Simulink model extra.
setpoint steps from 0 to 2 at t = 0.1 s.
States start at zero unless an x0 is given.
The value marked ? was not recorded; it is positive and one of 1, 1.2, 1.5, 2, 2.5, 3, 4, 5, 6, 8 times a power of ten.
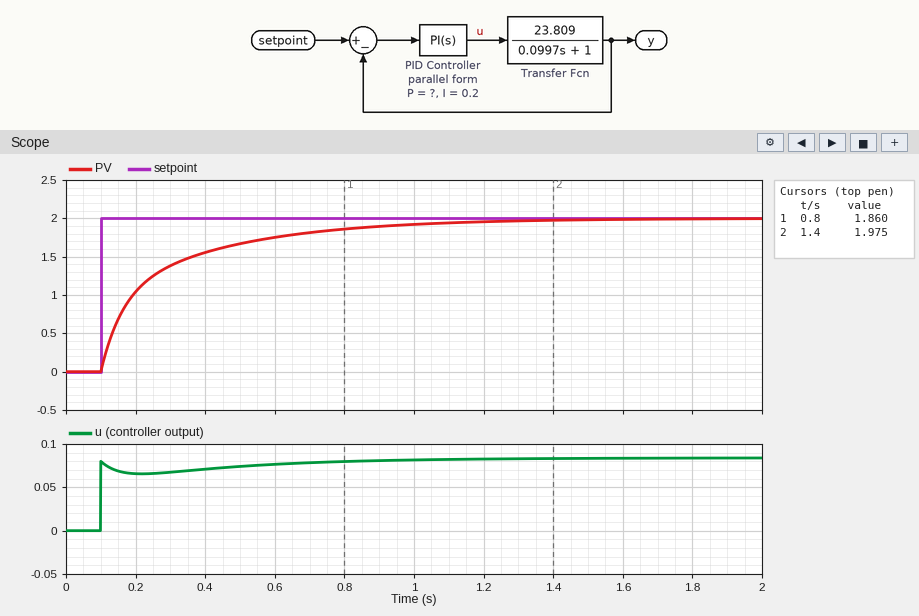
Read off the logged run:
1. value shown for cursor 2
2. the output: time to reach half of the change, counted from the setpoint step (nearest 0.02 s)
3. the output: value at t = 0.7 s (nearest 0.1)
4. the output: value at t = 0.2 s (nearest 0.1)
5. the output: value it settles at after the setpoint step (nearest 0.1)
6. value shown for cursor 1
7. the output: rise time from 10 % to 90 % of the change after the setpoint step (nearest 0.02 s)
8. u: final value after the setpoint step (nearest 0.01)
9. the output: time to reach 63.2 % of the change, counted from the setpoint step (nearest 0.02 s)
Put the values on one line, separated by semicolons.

1.975; 0.10 s; 1.8; 1.0; 2.0; 1.860; 0.56 s; 0.08; 0.16 s
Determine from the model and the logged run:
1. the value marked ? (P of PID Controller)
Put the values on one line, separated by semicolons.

0.04
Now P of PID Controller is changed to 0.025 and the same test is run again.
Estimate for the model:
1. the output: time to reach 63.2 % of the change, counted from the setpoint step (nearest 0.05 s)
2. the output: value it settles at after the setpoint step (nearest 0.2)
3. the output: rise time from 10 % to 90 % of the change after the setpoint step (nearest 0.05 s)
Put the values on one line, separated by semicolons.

0.20 s; 2.0; 0.50 s
